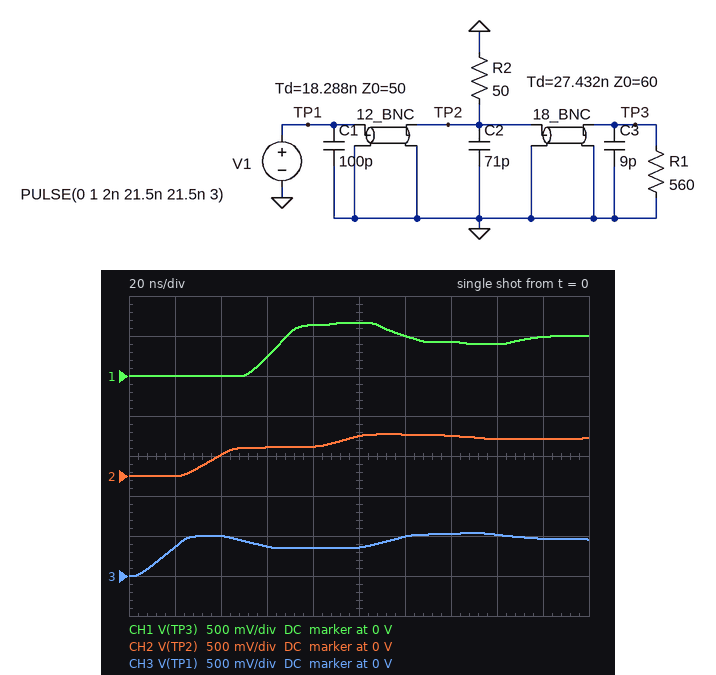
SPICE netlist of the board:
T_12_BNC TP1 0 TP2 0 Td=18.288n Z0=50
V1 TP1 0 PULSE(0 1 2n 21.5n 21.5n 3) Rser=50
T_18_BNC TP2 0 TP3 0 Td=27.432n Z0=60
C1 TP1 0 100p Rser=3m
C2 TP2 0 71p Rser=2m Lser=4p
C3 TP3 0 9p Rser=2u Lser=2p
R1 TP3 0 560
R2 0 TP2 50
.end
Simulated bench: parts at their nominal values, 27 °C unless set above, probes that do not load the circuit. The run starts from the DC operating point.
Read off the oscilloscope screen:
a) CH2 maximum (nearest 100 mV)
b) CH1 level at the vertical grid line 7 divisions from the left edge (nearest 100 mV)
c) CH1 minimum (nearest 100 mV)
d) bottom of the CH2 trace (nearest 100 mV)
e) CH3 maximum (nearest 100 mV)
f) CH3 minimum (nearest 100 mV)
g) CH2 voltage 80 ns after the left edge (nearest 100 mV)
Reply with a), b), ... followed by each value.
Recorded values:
a) 500 mV
b) 400 mV
c) 0 V
d) 0 V
e) 500 mV
f) 0 V
g) 400 mV
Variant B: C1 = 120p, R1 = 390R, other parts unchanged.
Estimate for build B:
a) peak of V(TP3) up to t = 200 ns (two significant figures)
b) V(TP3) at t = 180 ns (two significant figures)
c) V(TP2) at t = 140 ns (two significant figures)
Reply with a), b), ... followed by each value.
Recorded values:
a) 640 mV
b) 470 mV
c) 490 mV
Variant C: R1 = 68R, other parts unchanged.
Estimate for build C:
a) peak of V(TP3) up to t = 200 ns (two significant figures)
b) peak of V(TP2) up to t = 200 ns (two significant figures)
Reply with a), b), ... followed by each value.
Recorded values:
a) 390 mV
b) 370 mV
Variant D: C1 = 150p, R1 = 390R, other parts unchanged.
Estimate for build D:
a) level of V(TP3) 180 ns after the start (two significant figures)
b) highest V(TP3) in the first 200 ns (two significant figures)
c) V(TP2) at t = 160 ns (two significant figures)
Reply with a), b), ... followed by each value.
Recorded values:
a) 470 mV
b) 640 mV
c) 460 mV
